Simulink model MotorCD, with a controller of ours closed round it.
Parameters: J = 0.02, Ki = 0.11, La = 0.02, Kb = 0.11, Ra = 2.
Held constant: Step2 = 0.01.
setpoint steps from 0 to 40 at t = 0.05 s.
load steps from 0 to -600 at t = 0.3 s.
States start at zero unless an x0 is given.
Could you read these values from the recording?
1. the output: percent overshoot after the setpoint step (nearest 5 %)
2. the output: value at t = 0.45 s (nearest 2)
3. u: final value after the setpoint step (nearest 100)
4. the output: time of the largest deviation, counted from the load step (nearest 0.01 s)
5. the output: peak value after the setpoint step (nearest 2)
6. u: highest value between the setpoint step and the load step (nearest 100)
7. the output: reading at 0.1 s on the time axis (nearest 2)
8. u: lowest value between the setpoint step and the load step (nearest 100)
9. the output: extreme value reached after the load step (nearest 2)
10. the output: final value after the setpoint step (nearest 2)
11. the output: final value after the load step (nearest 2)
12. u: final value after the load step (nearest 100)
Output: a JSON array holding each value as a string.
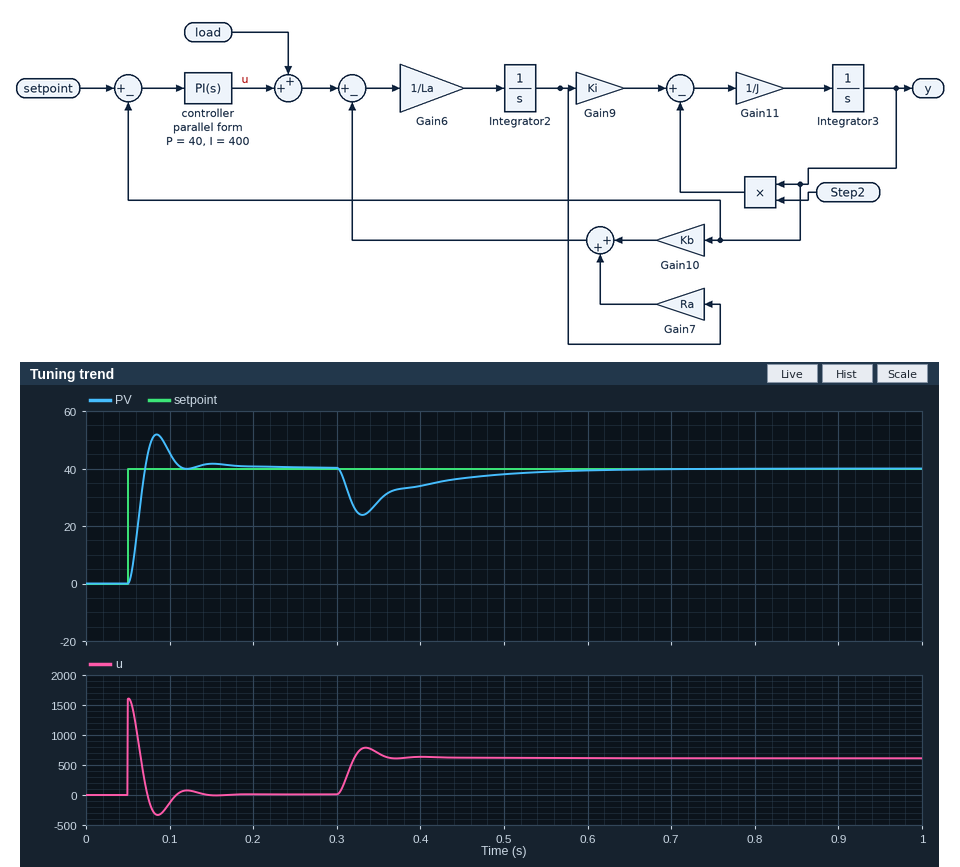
["30 %", "36", "0", "0.03 s", "52", "1600", "46", "-300", "24", "40", "40", "600"]
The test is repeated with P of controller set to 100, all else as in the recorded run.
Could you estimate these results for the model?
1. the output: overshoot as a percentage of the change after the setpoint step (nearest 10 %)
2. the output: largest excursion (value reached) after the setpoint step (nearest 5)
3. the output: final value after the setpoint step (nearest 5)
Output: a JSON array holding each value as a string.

["40 %", "55", "40"]
